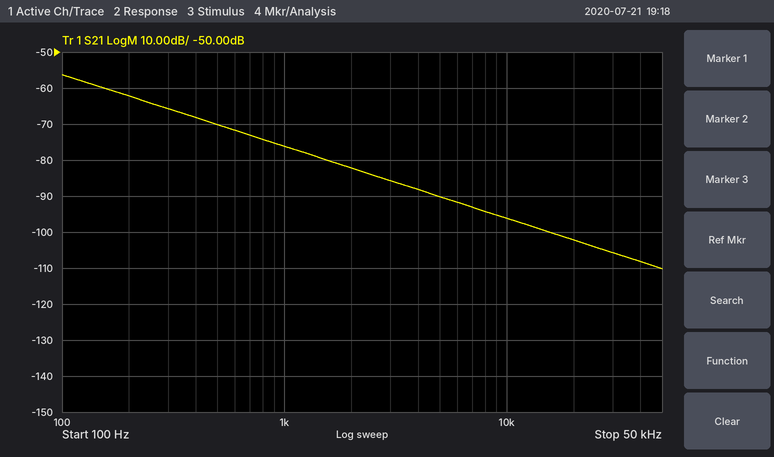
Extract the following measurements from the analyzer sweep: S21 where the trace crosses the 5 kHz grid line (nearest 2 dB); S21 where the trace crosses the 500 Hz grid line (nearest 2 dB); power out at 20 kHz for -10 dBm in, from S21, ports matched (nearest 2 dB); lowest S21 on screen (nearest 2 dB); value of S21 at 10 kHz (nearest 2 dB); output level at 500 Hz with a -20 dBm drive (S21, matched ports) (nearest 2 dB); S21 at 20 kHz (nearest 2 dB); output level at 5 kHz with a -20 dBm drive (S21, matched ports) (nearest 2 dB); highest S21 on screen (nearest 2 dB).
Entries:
-90 dB
-70 dB
-112 dBm
-110 dB
-96 dB
-90 dBm
-102 dB
-110 dBm
-56 dB
